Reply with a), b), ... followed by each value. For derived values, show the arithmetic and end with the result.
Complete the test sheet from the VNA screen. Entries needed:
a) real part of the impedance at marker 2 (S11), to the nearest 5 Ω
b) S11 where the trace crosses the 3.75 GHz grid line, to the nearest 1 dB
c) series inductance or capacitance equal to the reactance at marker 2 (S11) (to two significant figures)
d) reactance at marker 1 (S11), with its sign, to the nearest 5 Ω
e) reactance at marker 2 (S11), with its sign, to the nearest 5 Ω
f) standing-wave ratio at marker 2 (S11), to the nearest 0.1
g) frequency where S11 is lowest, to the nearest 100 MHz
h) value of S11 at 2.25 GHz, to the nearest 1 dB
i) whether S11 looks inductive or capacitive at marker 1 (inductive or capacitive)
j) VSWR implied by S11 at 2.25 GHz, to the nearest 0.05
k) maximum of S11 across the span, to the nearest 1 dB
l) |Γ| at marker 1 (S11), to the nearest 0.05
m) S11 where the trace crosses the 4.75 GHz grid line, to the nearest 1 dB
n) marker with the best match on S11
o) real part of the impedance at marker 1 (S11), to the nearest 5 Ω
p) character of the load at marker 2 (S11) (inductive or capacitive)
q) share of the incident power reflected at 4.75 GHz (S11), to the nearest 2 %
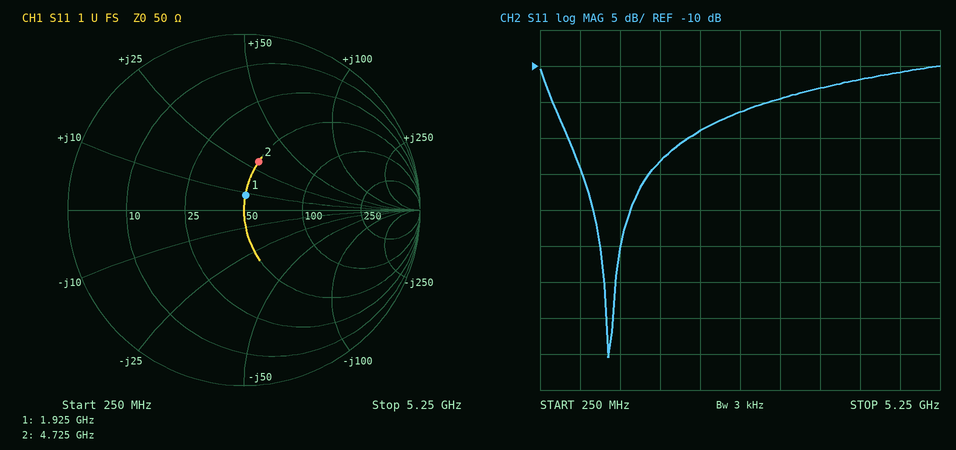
a) 50 Ω
b) -13 dB
c) L = 30 Ω/(2π × 4.725 GHz) ≈ 1.0 nH
d) +10 Ω
e) +30 Ω
f) 1.8
g) 1.1 GHz
h) -19 dB
i) inductive
j) |Γ| = 10^(-19/20) = 0.1122; VSWR = (1 + 0.1122)/(1 − 0.1122) ≈ 1.25
k) -10 dB
l) 0.10
m) -11 dB
n) marker 1
o) 50 Ω
p) inductive
q) 10^(-11/10) ≈ 8 %
